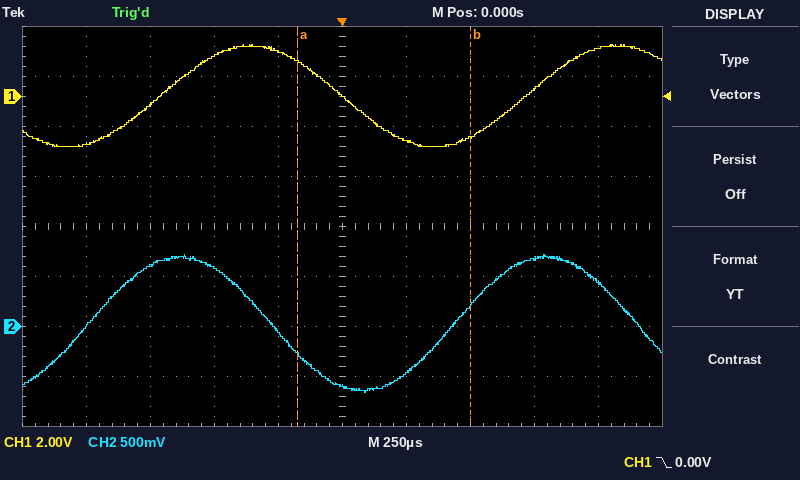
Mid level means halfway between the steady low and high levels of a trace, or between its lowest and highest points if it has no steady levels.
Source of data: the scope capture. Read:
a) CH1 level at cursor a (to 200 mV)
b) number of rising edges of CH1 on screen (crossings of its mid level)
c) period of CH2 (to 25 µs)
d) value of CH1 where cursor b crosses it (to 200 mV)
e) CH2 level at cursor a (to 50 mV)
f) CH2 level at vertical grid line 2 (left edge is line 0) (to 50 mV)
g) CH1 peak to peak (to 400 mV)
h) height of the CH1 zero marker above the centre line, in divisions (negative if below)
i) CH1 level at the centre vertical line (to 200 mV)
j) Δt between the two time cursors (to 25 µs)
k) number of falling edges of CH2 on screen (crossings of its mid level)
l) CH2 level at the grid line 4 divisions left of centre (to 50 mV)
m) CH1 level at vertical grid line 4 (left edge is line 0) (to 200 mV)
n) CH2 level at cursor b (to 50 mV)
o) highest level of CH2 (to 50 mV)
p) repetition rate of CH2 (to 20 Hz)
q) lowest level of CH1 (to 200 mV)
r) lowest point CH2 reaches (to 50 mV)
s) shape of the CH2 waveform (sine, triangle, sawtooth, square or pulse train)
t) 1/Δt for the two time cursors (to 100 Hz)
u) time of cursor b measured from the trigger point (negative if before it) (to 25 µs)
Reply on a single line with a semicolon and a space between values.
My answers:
1.4 V; 2; 1.425 ms; -1.6 V; -300 mV; 600 mV; 4.0 V; +2.6 div; 0.0 V; 675 µs; 2; 0 mV; 1.8 V; 200 mV; 700 mV; 700 Hz; -2.0 V; -650 mV; sine; 1.5 kHz; +500 µs
